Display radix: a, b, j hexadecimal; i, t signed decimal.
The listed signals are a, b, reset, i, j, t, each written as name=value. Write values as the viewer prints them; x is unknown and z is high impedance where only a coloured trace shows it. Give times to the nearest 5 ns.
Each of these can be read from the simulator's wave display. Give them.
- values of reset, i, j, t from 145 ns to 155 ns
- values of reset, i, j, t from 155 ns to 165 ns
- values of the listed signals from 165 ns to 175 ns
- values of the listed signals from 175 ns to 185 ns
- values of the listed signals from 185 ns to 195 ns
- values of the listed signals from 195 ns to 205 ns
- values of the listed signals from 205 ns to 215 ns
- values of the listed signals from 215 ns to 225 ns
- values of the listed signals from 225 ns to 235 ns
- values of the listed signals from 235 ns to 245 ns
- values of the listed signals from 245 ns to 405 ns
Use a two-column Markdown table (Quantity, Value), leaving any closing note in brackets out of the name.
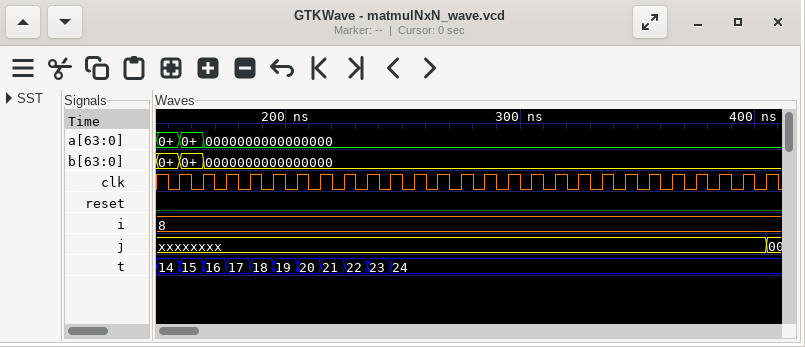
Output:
| Quantity | Value |
|---|---|
| values of reset, i, j, t from 145 ns to 155 ns | reset=0, i=8, j=xxxxxxxx, t=14 |
| values of reset, i, j, t from 155 ns to 165 ns | reset=0, i=8, j=xxxxxxxx, t=15 |
| values of the listed signals from 165 ns to 175 ns | a=0000000000000000, b=0000000000000000, reset=0, i=8, j=xxxxxxxx, t=16 |
| values of the listed signals from 175 ns to 185 ns | a=0000000000000000, b=0000000000000000, reset=0, i=8, j=xxxxxxxx, t=17 |
| values of the listed signals from 185 ns to 195 ns | a=0000000000000000, b=0000000000000000, reset=0, i=8, j=xxxxxxxx, t=18 |
| values of the listed signals from 195 ns to 205 ns | a=0000000000000000, b=0000000000000000, reset=0, i=8, j=xxxxxxxx, t=19 |
| values of the listed signals from 205 ns to 215 ns | a=0000000000000000, b=0000000000000000, reset=0, i=8, j=xxxxxxxx, t=20 |
| values of the listed signals from 215 ns to 225 ns | a=0000000000000000, b=0000000000000000, reset=0, i=8, j=xxxxxxxx, t=21 |
| values of the listed signals from 225 ns to 235 ns | a=0000000000000000, b=0000000000000000, reset=0, i=8, j=xxxxxxxx, t=22 |
| values of the listed signals from 235 ns to 245 ns | a=0000000000000000, b=0000000000000000, reset=0, i=8, j=xxxxxxxx, t=23 |
| values of the listed signals from 245 ns to 405 ns | a=0000000000000000, b=0000000000000000, reset=0, i=8, j=xxxxxxxx, t=24 |
